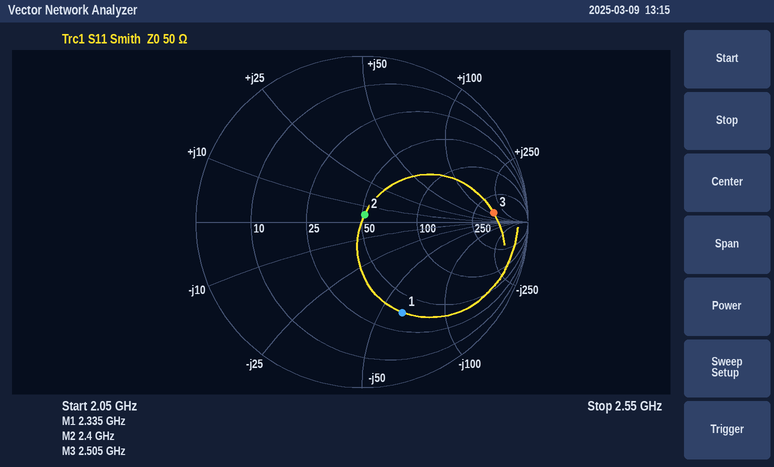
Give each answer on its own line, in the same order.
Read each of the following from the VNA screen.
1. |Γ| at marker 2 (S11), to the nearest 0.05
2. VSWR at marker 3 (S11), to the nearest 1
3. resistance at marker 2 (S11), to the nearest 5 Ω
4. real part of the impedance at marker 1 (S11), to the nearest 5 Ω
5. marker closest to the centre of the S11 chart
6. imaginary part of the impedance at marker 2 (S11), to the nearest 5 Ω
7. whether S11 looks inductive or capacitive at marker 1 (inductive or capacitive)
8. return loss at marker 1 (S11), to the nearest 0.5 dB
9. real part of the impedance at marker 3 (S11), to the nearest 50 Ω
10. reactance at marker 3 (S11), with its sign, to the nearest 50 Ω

0.05
9
50 Ω
35 Ω
marker 2
+5 Ω
capacitive
4.5 dB
400 Ω
+100 Ω
